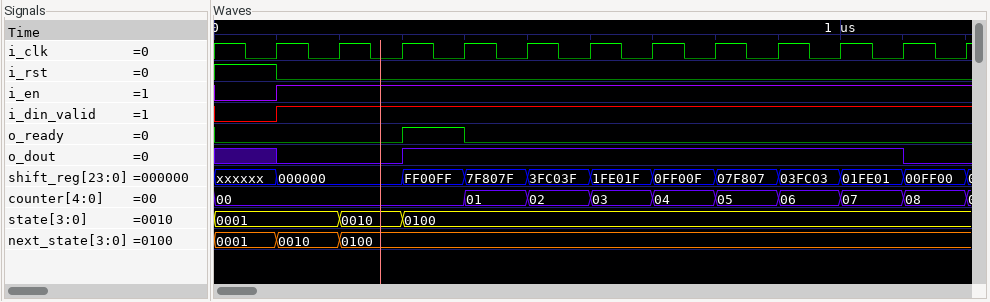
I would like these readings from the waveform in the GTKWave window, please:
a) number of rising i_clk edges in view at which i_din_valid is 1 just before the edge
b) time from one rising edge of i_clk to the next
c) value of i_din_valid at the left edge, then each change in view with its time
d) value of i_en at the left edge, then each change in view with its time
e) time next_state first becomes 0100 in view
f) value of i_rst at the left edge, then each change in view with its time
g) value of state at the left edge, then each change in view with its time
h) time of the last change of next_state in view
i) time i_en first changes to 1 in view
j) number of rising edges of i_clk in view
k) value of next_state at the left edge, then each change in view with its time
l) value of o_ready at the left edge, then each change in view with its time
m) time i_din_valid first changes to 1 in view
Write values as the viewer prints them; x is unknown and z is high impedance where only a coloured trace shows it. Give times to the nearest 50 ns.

11
100 ns
0, 1 at 100 ns
0, 1 at 100 ns
200 ns
1, 0 at 100 ns
0001, 0010 at 200 ns, 0100 at 300 ns
200 ns
100 ns
12
0001, 0010 at 100 ns, 0100 at 200 ns
0, 1 at 300 ns, 0 at 400 ns
100 ns
